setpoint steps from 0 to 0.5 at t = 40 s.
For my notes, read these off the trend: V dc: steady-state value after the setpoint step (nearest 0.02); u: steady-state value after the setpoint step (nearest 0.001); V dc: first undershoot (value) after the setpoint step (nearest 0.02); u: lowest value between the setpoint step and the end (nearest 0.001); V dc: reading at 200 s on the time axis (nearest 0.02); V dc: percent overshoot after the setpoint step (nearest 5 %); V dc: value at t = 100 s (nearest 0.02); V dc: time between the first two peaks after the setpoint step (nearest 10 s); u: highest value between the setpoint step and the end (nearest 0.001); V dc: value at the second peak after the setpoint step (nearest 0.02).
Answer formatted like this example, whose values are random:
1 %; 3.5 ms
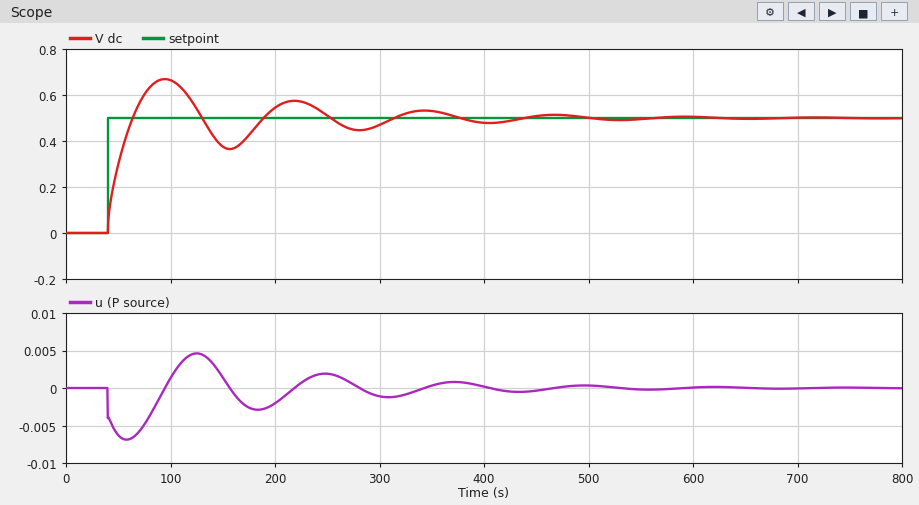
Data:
0.50; 0.000; 0.36; -0.007; 0.54; 35 %; 0.66; 120 s; 0.005; 0.58
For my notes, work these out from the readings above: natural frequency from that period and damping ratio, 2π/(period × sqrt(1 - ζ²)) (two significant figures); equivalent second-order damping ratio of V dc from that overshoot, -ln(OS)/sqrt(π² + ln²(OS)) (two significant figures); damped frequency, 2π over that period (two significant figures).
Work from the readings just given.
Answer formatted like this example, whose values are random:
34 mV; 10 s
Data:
0.055 rad/s; 0.32; 0.052 rad/s
